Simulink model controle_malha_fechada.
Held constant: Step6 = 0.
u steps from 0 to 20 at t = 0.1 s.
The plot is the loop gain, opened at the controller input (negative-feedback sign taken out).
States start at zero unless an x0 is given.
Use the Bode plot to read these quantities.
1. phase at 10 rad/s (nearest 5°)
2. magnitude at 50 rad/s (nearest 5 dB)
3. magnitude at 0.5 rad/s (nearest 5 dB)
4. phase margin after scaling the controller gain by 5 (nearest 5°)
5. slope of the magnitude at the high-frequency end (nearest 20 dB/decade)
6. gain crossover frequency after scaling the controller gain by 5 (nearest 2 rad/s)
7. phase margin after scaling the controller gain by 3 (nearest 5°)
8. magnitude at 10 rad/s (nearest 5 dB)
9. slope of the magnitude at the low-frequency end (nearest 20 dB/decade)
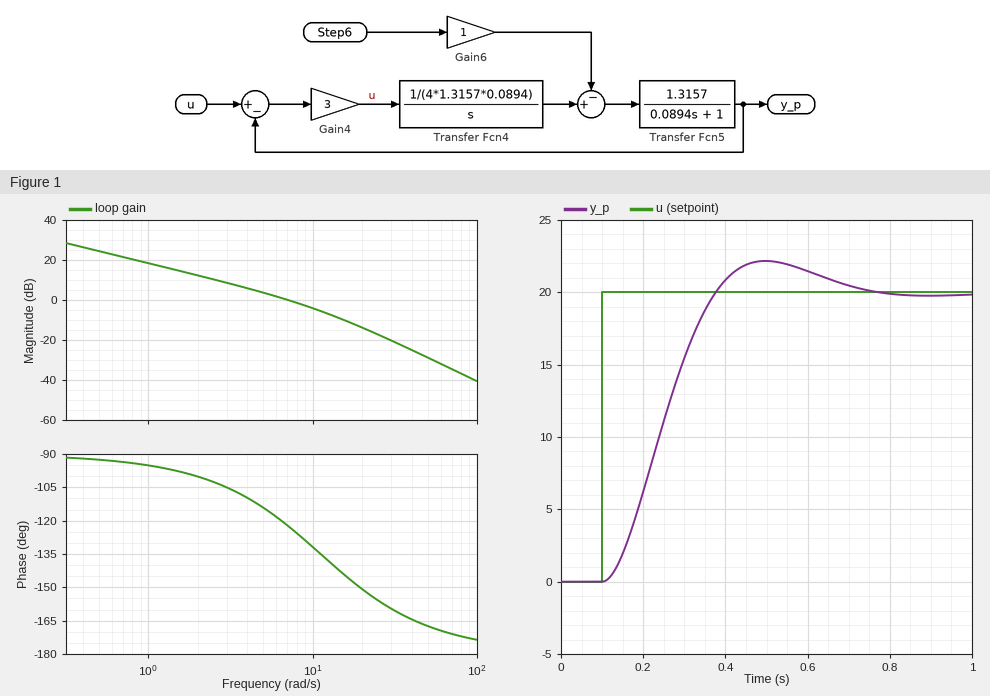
-130°
-30 dB
25 dB
30°
-40 dB/decade
20 rad/s
35°
-5 dB
-20 dB/decade
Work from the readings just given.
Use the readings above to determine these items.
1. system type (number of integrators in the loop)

1
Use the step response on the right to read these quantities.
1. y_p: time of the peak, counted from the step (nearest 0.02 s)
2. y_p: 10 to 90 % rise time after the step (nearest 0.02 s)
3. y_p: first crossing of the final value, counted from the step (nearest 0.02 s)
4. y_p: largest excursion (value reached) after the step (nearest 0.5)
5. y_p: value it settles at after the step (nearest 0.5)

0.40 s
0.18 s
0.28 s
22.0
20.0
